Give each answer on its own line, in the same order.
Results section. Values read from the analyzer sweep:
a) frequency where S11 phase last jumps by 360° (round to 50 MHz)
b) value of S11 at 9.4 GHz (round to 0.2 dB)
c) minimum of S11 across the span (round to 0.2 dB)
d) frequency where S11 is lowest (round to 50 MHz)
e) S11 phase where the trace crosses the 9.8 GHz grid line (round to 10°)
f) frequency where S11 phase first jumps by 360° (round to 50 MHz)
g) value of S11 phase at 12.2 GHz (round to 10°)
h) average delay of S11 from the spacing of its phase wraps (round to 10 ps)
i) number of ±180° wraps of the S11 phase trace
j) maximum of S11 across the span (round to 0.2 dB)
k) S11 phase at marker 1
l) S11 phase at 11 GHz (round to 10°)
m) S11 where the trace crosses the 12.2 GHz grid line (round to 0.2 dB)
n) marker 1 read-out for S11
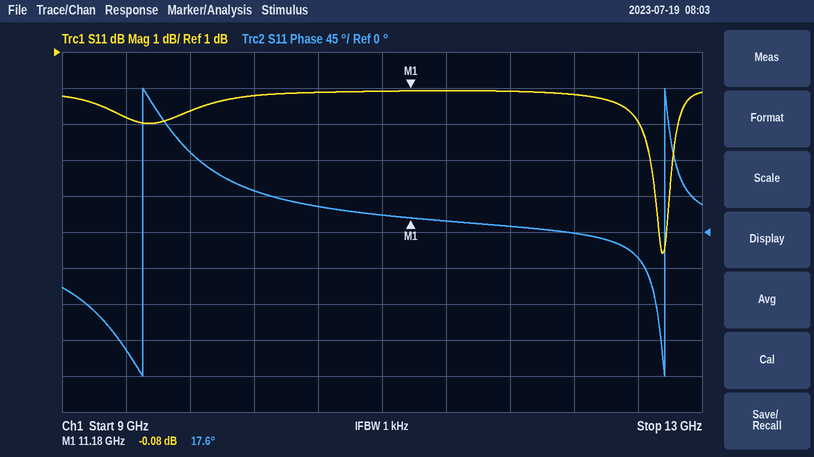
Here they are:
12.75 GHz
-0.8 dB
-4.6 dB
12.75 GHz
100°
9.50 GHz
0°
310 ps
2
0.0 dB
17.6°
20°
-0.2 dB
-0.08 dB
